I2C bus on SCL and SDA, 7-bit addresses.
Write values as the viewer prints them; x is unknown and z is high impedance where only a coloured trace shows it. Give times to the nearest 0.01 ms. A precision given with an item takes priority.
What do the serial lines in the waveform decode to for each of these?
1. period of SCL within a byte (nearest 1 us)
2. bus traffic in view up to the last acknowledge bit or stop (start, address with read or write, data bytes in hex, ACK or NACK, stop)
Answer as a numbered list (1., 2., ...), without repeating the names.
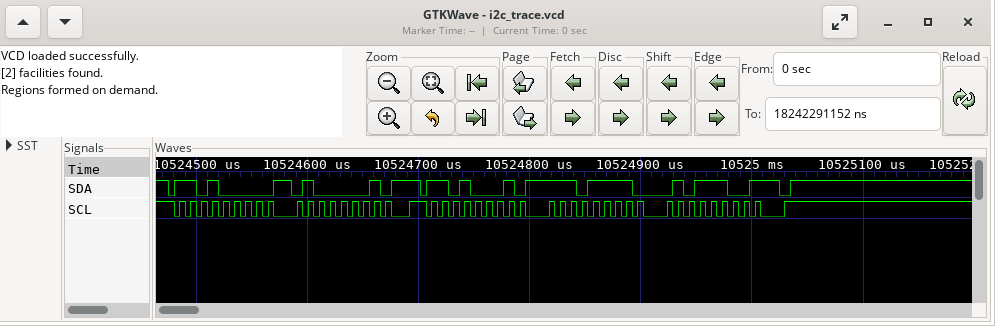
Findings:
1. 10 us
2. start, address 68 write ACK, 41 ACK, repeated start, address 68 read ACK, EF ACK, 5C NACK, stop
